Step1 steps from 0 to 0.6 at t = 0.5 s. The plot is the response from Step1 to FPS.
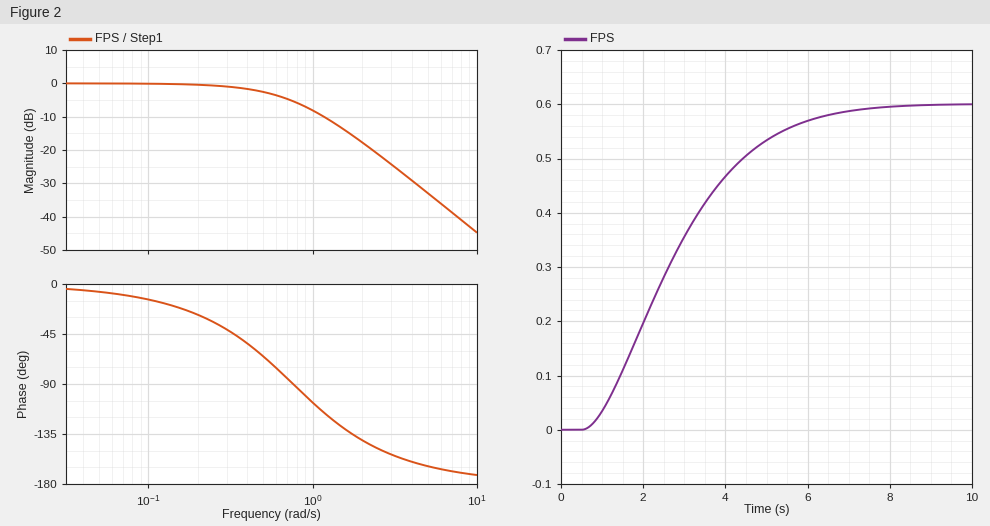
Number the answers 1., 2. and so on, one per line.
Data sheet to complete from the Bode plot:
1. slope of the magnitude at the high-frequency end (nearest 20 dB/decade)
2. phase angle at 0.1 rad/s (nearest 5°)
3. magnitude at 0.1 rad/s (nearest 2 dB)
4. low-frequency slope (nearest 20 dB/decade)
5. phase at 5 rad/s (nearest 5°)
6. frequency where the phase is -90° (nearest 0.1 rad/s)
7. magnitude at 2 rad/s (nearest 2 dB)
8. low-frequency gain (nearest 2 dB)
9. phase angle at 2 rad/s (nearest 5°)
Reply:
1. -40 dB/decade
2. -15°
3. 0 dB
4. 0 dB/decade
5. -165°
6. 0.8 rad/s
7. -18 dB
8. 0 dB
9. -140°
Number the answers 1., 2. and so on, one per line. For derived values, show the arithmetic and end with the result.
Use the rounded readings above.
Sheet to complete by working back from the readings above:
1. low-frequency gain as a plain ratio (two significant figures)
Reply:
1. 10^(0 / 20) = 1.0
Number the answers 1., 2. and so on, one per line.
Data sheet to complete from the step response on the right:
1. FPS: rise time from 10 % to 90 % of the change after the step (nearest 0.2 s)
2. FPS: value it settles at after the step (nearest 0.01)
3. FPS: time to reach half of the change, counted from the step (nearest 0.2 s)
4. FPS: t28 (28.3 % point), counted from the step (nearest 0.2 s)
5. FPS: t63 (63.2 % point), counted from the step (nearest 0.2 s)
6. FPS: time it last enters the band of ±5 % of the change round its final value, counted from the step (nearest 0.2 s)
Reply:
1. 4.0 s
2. 0.60
3. 2.2 s
4. 1.4 s
5. 2.6 s
6. 5.6 s
